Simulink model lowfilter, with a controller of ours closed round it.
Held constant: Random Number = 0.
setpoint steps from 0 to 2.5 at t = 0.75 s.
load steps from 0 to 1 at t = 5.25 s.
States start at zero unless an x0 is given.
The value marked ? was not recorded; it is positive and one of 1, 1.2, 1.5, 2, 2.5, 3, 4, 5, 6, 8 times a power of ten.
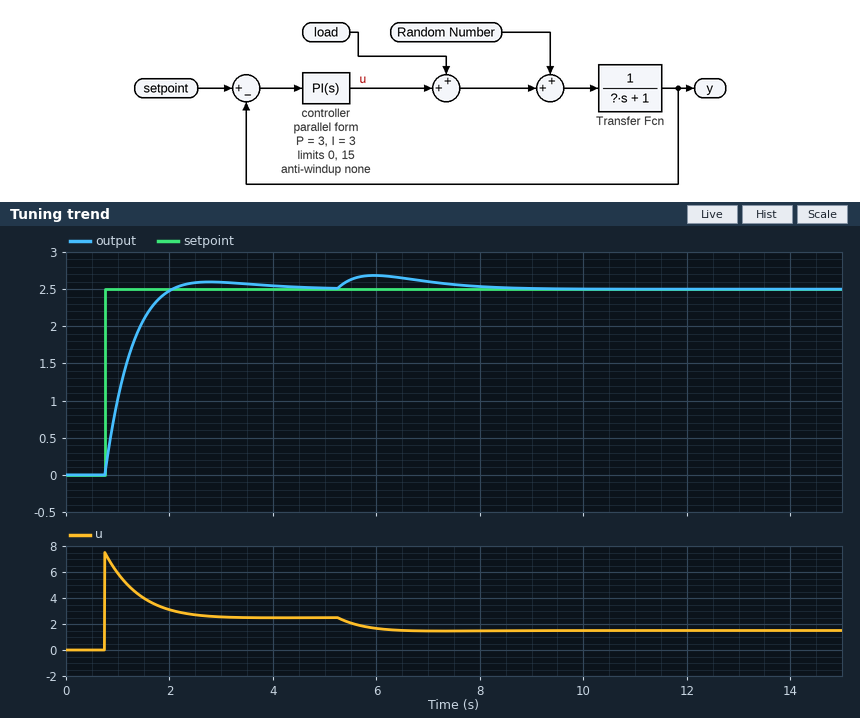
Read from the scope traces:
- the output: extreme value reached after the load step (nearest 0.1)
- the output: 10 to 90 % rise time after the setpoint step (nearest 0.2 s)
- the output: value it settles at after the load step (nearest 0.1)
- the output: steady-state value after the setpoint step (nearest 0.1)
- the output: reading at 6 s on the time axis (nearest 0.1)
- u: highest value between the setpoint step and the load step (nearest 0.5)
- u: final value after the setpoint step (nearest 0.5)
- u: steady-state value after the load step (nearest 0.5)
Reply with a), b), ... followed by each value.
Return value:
a) 2.7
b) 0.8 s
c) 2.5
d) 2.5
e) 2.7
f) 7.5
g) 2.5
h) 1.5
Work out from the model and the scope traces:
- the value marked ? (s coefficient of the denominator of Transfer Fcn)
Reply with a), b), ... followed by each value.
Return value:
a) 1.5
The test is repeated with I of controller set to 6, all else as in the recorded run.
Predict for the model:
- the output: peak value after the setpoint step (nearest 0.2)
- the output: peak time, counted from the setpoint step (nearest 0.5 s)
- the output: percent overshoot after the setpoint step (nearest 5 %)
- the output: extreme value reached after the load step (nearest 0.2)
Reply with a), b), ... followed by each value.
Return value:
a) 2.8
b) 1.5 s
c) 15 %
d) 2.6
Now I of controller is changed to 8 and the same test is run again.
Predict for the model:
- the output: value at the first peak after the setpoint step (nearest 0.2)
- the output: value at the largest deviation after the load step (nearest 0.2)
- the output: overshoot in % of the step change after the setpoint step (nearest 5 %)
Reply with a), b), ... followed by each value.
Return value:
a) 3.0
b) 2.6
c) 20 %
